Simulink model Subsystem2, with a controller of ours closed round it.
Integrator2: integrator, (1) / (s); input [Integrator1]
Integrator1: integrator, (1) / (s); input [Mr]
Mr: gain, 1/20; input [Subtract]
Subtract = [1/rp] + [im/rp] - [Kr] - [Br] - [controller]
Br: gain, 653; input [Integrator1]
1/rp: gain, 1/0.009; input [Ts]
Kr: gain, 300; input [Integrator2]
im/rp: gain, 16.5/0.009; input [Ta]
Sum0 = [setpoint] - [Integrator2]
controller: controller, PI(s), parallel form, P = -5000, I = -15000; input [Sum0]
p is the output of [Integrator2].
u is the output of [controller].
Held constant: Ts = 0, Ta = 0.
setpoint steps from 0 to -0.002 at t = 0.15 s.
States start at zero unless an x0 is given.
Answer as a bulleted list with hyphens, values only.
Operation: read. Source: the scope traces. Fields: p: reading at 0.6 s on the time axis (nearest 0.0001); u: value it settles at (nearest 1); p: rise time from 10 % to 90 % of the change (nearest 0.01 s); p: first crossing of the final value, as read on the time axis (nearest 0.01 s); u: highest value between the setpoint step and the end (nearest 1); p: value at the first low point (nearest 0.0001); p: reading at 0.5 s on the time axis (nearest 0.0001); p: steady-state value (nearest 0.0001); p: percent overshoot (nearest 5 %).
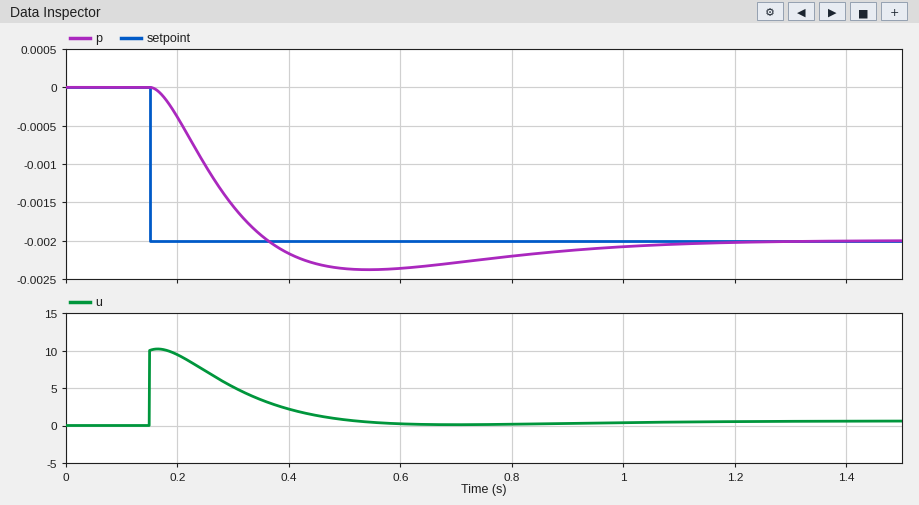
- -0.0024
- 1
- 0.15 s
- 0.36 s
- 10
- -0.0024
- -0.0024
- -0.0020
- 20 %
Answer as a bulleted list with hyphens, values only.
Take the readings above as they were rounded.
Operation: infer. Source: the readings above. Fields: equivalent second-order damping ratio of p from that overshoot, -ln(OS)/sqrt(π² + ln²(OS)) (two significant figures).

- 0.46
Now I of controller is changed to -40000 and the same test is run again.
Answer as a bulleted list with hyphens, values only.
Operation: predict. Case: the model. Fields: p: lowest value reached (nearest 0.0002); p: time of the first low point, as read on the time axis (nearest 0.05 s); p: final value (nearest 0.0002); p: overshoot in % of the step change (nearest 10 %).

- -0.0028
- 0.45 s
- -0.0020
- 40 %
